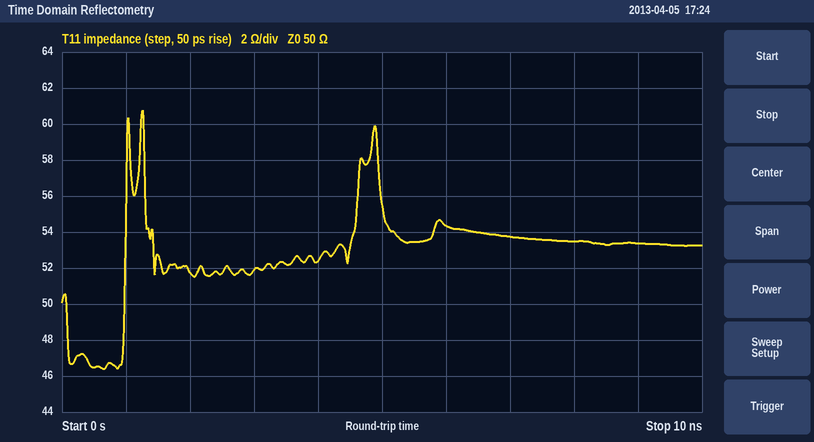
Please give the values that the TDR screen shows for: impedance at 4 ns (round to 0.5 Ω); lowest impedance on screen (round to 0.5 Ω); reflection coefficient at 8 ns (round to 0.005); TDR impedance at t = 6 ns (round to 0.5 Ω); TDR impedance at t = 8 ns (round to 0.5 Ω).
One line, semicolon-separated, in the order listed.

52.5 Ω; 46.5 Ω; +0.035; 54.5 Ω; 53.5 Ω
